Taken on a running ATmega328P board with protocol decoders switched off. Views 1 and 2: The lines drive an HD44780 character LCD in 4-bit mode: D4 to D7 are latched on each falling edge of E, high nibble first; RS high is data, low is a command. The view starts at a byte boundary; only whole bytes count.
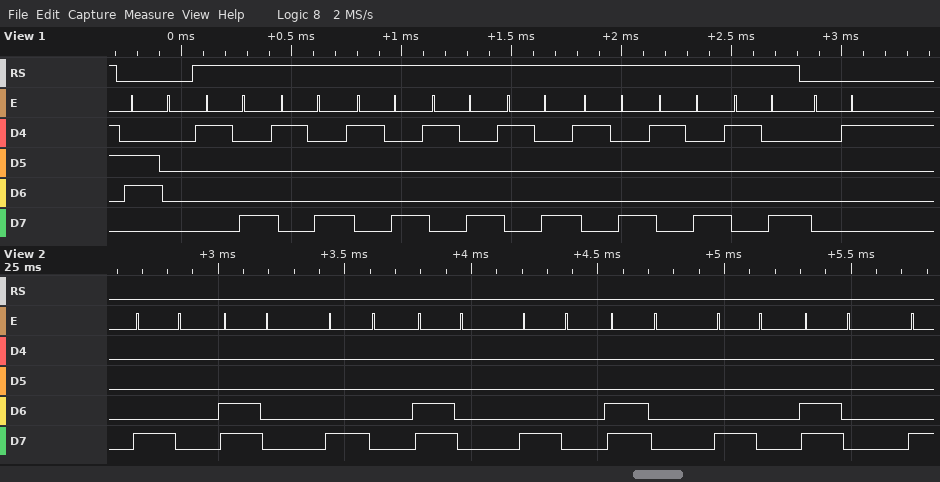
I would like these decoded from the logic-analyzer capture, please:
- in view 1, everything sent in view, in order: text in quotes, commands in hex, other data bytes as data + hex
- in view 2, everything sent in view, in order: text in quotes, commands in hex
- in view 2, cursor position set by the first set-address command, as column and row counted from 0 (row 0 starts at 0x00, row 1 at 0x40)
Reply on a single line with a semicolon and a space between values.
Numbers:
0x60 data 18 18 18 18 18 18 18 18 0x01; 0x80 0xC0 0x80 0xC0 0x80 0xC0 0x80 0xC0; column 0, row 0
